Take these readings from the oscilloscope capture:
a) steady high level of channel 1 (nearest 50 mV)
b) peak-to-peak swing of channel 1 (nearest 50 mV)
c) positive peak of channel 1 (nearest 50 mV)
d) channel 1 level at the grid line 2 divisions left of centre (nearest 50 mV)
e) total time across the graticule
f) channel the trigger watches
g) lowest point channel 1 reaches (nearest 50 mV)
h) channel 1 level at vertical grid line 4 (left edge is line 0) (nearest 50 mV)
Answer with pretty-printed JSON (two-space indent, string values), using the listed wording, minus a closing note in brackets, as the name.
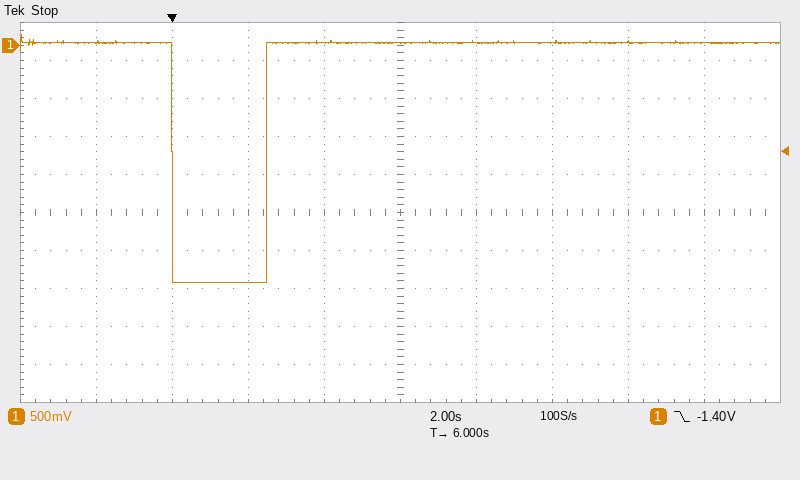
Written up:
{
  "steady high level of channel 1": "50 mV",
  "peak-to-peak swing of channel 1": "3.25 V",
  "positive peak of channel 1": "150 mV",
  "channel 1 level at the grid line 2 divisions left of centre": "-3.10 V",
  "total time across the graticule": "20 s",
  "channel the trigger watches": "channel 1",
  "lowest point channel 1 reaches": "-3.10 V",
  "channel 1 level at vertical grid line 4 (left edge is line 0)": "50 mV"
}
